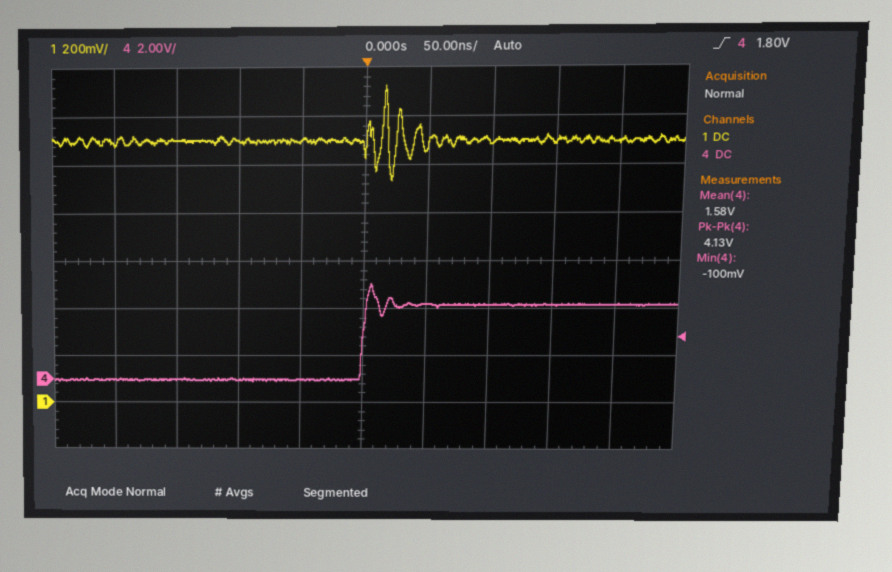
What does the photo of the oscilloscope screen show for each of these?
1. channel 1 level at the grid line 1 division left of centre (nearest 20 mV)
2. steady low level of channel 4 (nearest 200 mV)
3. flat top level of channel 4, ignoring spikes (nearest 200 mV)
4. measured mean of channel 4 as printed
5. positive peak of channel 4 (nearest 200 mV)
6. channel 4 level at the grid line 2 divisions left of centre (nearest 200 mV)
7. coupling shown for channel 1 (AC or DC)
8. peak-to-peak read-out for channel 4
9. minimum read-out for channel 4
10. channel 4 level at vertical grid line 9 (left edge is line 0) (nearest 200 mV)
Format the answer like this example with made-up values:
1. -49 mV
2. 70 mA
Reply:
1. 1.10 V
2. 0.0 V
3. 3.2 V
4. 1.58 V
5. 4.0 V
6. 0.0 V
7. DC
8. 4.13 V
9. -100 mV
10. 3.2 V
